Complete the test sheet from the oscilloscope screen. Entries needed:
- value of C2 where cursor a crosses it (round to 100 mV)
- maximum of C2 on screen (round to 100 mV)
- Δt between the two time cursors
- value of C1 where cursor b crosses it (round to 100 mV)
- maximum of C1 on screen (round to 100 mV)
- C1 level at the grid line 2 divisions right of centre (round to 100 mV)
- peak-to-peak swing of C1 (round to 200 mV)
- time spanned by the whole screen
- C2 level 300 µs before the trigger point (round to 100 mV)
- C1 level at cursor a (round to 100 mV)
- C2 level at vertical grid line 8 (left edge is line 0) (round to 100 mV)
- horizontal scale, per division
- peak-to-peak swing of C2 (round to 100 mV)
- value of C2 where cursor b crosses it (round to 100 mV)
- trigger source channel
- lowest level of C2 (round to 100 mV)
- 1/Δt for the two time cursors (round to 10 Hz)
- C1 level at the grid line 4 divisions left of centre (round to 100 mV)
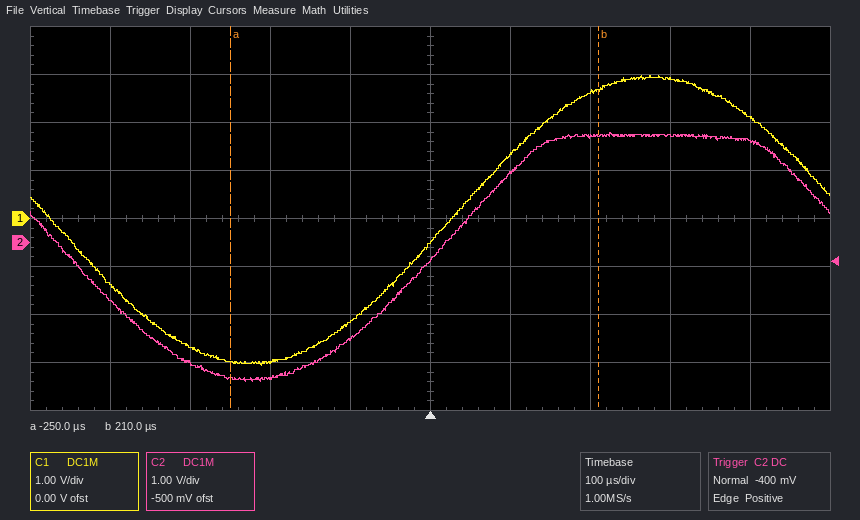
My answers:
-2.8 V
2.3 V
460 µs
2.7 V
3.0 V
2.6 V
6.0 V
1 ms
-2.5 V
-3.0 V
2.2 V
100 µs
5.2 V
2.2 V
C2
-2.9 V
2.17 kHz
-1.4 V
